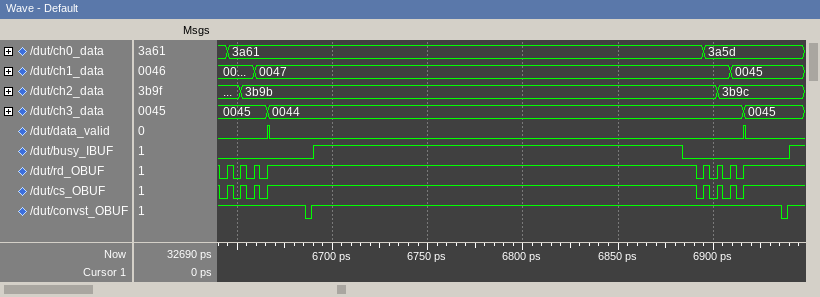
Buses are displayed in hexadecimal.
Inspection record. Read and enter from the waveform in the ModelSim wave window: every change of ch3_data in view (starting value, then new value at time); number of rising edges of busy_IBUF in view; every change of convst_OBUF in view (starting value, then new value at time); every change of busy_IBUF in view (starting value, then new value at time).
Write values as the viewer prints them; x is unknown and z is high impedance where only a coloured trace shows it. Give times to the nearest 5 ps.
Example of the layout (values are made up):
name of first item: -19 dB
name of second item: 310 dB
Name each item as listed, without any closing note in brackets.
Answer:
every change of ch3_data in view: 0045, 0044 at 6665 ps, 0045 at 6915 ps
number of rising edges of busy_IBUF in view: 2
every change of convst_OBUF in view: 1, 0 at 6685 ps, 1 at 6690 ps, 0 at 6935 ps, 1 at 6940 ps
every change of busy_IBUF in view: 0, 1 at 6690 ps, 0 at 6885 ps, 1 at 6940 ps
